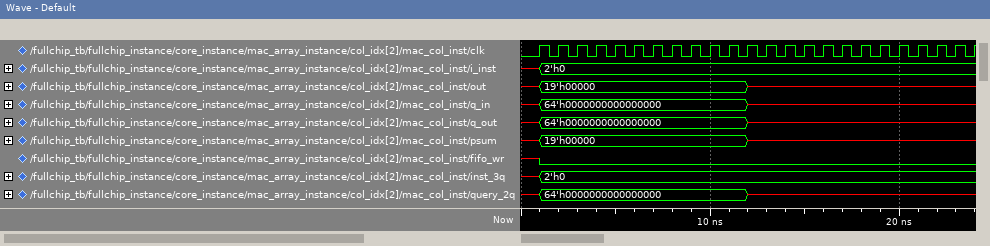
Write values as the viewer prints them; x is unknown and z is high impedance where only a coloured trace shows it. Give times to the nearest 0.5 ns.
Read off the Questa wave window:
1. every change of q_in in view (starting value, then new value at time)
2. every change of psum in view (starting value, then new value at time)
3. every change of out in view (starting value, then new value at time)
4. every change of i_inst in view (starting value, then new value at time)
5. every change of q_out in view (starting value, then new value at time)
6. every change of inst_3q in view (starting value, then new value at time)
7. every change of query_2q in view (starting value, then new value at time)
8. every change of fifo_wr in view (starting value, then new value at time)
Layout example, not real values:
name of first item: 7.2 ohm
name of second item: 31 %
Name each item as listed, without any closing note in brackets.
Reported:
every change of q_in in view: x, 64'h0000000000000000 at 1 ns, x at 12 ns
every change of psum in view: x, 19'h00000 at 1 ns, x at 12 ns
every change of out in view: x, 19'h00000 at 1 ns, x at 12 ns
every change of i_inst in view: x, 2'h0 at 1 ns
every change of q_out in view: x, 64'h0000000000000000 at 1 ns, x at 12 ns
every change of inst_3q in view: x, 2'h0 at 1 ns
every change of query_2q in view: x, 64'h0000000000000000 at 1 ns, x at 12 ns
every change of fifo_wr in view: x, 0 at 1 ns
